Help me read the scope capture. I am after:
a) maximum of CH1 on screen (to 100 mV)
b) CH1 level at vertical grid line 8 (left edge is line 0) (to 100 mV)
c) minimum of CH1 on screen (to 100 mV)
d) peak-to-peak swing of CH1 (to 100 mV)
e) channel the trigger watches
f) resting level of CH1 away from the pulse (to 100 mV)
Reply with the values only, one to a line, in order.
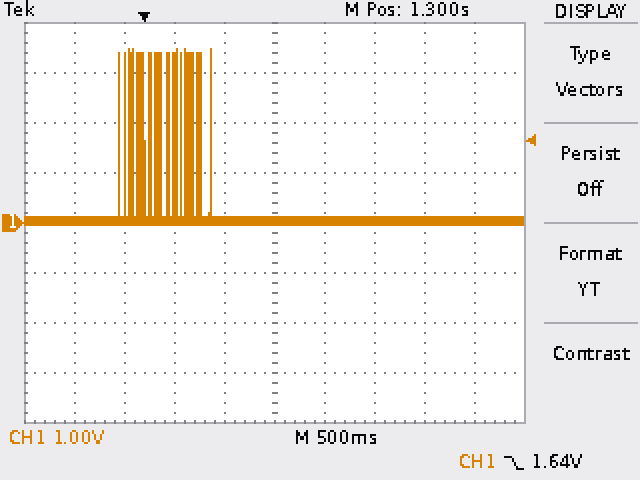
3.5 V
0.0 V
0.0 V
3.5 V
CH1
0.0 V
